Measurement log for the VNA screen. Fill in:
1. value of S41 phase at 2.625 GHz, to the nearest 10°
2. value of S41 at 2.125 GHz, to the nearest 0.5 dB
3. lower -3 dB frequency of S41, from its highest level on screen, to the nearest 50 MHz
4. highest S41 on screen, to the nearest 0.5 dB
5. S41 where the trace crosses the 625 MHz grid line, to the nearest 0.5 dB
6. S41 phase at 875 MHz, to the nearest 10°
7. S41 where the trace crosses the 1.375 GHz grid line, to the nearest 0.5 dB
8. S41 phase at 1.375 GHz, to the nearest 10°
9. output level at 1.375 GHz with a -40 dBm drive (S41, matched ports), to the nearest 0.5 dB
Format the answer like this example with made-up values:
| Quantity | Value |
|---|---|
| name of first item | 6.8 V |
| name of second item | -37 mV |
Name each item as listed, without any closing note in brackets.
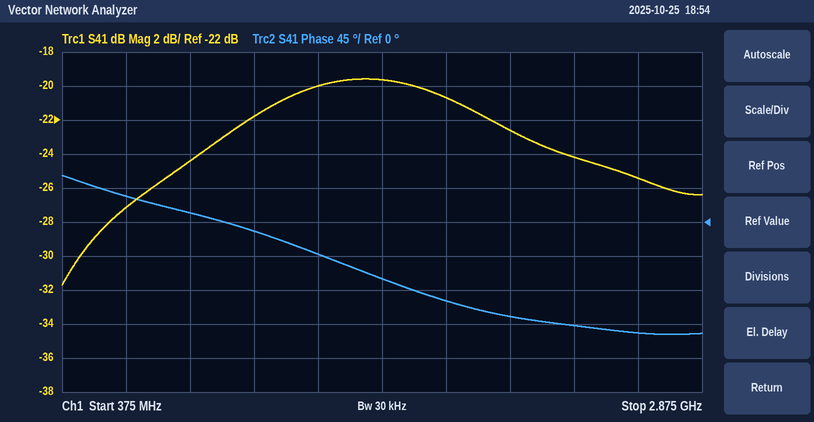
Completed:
| Quantity | Value |
|---|---|
| value of S41 phase at 2.625 GHz, to the nearest 10° | -150° |
| value of S41 at 2.125 GHz, to the nearest 0.5 dB | -22.5 dB |
| lower -3 dB frequency of S41, from its highest level on screen, to the nearest 50 MHz | 1.05 GHz |
| highest S41 on screen, to the nearest 0.5 dB | -19.5 dB |
| S41 where the trace crosses the 625 MHz grid line, to the nearest 0.5 dB | -27.0 dB |
| S41 phase at 875 MHz, to the nearest 10° | 10° |
| S41 where the trace crosses the 1.375 GHz grid line, to the nearest 0.5 dB | -20.0 dB |
| S41 phase at 1.375 GHz, to the nearest 10° | -40° |
| output level at 1.375 GHz with a -40 dBm drive (S41, matched ports), to the nearest 0.5 dB | -60.0 dBm |
